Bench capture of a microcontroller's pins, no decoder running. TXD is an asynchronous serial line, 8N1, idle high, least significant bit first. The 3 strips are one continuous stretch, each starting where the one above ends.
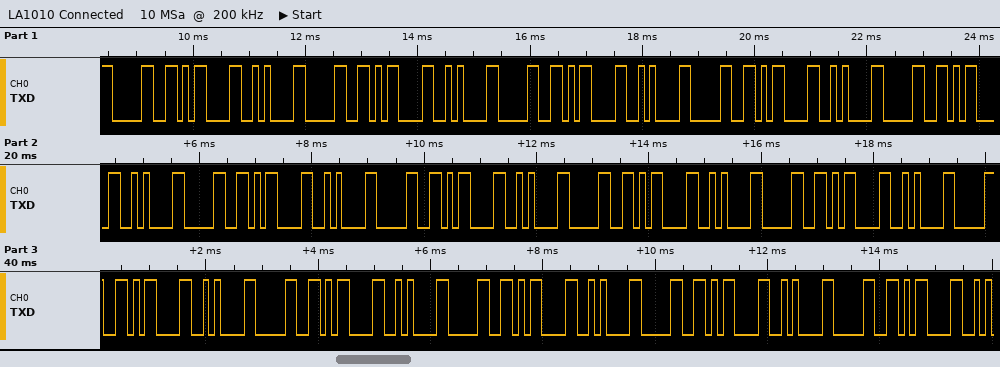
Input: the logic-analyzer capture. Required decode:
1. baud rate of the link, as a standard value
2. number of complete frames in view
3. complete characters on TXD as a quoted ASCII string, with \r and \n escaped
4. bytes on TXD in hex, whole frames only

9600 baud
41
"0\r\n0\r\n0\r\n0\r\n0\r\n0\r\n0\r\n0\r\n0\r\n0\r\n0\r\n0\r\n0\r\n0\r"
30 0D 0A 30 0D 0A 30 0D 0A 30 0D 0A 30 0D 0A 30 0D 0A 30 0D 0A 30 0D 0A 30 0D 0A 30 0D 0A 30 0D 0A 30 0D 0A 30 0D 0A 30 0D
